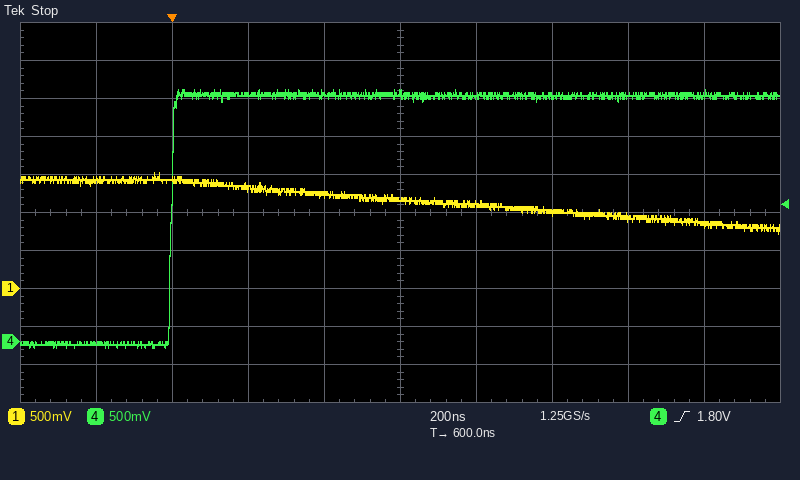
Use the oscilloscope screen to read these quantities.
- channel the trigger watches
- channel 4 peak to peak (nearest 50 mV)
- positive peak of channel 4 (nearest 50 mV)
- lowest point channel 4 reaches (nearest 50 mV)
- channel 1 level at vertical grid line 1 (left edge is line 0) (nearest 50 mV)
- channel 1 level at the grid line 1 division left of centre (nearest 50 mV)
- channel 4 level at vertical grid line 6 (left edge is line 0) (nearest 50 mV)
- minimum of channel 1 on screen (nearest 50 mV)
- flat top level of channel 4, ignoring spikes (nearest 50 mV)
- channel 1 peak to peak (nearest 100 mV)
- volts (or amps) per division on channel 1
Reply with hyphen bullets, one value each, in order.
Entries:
- channel 4
- 3.40 V
- 3.30 V
- -100 mV
- 1.45 V
- 1.25 V
- 3.25 V
- 700 mV
- 3.25 V
- 800 mV
- 500 mV
